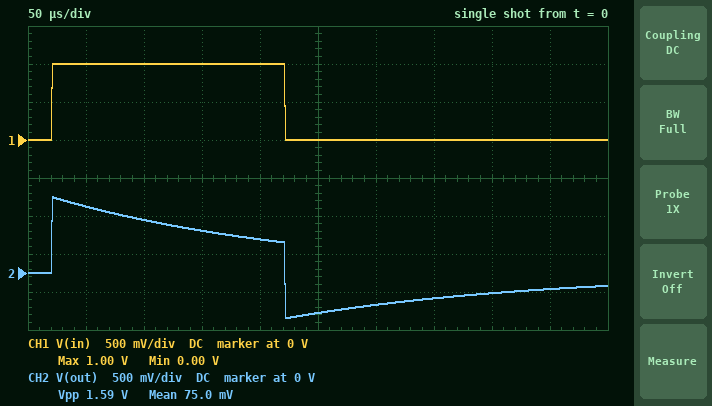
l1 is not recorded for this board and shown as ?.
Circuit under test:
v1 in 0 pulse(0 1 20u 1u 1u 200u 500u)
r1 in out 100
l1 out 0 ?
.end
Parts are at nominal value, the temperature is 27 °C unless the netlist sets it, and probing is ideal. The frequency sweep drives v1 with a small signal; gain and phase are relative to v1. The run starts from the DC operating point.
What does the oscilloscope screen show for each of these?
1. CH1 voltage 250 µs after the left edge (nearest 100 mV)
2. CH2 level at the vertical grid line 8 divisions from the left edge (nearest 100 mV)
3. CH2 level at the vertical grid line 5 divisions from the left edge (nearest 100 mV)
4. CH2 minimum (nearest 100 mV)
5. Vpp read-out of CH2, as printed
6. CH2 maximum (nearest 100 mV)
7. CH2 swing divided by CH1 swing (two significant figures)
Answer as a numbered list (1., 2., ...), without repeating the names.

1. 0 V
2. -300 mV
3. -500 mV
4. -600 mV
5. 1.59 V
6. 1.0 V
7. 1.6
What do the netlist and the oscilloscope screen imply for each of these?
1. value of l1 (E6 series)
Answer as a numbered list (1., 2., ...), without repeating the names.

1. 22 mH
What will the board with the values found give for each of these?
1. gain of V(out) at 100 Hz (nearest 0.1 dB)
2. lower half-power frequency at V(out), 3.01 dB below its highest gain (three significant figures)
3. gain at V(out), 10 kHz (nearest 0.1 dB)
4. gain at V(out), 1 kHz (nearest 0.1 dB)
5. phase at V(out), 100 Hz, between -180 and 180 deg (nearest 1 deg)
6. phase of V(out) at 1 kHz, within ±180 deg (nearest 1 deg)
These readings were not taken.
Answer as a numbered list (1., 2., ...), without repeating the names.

1. -17.3 dB
2. 723 Hz
3. 0 dB
4. -1.8 dB
5. 82 deg
6. 36 deg
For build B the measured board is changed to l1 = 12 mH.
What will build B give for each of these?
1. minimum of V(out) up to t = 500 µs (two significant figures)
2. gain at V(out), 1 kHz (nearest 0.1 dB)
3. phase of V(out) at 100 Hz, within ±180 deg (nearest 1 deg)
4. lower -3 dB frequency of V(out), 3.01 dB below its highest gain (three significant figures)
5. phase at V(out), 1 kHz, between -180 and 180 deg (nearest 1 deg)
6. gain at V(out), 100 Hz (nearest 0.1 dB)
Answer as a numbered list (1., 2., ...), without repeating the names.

1. -810 mV
2. -4.4 dB
3. 86 deg
4. 1.33 kHz
5. 53 deg
6. -22.5 dB
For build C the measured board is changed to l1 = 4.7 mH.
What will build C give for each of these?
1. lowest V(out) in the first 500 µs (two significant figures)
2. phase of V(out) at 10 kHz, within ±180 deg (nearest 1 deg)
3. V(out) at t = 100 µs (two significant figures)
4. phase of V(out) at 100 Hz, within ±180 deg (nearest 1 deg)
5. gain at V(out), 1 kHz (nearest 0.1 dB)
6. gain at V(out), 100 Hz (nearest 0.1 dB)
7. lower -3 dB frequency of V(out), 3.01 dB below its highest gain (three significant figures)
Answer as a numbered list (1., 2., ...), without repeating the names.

1. -980 mV
2. 19 deg
3. 180 mV
4. 88 deg
5. -11.0 dB
6. -30.6 dB
7. 3.39 kHz
